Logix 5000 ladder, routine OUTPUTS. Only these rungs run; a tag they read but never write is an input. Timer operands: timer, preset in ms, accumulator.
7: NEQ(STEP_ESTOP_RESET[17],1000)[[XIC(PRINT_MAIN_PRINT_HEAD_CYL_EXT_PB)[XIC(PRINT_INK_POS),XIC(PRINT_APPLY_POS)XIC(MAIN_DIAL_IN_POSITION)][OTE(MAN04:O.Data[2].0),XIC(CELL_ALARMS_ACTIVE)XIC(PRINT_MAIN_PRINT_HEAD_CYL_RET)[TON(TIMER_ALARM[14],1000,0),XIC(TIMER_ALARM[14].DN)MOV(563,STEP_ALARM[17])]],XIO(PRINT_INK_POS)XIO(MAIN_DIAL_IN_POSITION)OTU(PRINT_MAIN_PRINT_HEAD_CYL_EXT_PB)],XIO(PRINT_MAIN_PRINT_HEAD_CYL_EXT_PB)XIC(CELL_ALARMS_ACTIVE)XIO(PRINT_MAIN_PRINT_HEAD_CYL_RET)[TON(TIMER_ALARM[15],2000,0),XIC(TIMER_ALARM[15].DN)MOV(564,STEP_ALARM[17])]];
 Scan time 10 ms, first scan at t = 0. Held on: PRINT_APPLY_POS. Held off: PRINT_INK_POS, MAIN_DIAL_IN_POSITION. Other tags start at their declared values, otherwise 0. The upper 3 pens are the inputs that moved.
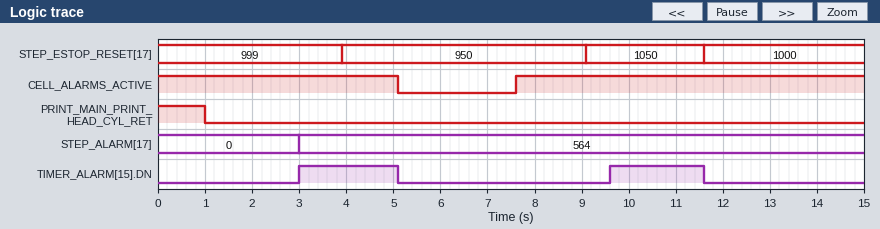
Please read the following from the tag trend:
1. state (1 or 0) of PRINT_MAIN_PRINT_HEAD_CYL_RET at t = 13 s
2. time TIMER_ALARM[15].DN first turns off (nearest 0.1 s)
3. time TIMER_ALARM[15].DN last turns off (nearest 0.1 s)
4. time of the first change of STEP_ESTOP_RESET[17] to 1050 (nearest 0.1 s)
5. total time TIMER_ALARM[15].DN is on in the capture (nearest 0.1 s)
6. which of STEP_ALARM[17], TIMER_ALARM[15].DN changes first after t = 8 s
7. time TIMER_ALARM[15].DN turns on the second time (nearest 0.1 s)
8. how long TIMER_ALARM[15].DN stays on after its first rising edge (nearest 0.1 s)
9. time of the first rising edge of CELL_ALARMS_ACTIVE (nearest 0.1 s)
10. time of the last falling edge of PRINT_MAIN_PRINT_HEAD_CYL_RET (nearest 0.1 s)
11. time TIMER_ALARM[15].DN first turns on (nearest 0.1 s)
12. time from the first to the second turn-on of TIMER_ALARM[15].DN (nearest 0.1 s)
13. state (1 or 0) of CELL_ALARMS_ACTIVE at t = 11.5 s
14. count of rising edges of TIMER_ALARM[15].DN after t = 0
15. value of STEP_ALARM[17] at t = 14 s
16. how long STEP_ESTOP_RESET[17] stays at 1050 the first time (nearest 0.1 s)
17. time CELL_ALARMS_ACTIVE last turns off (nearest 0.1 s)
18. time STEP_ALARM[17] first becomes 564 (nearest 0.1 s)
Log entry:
0
5.1 s
11.6 s
9.1 s
4.1 s
TIMER_ALARM[15].DN
9.6 s
2.1 s
7.6 s
1.0 s
3.0 s
6.6 s
1
2
564
2.5 s
5.1 s
3.0 s
